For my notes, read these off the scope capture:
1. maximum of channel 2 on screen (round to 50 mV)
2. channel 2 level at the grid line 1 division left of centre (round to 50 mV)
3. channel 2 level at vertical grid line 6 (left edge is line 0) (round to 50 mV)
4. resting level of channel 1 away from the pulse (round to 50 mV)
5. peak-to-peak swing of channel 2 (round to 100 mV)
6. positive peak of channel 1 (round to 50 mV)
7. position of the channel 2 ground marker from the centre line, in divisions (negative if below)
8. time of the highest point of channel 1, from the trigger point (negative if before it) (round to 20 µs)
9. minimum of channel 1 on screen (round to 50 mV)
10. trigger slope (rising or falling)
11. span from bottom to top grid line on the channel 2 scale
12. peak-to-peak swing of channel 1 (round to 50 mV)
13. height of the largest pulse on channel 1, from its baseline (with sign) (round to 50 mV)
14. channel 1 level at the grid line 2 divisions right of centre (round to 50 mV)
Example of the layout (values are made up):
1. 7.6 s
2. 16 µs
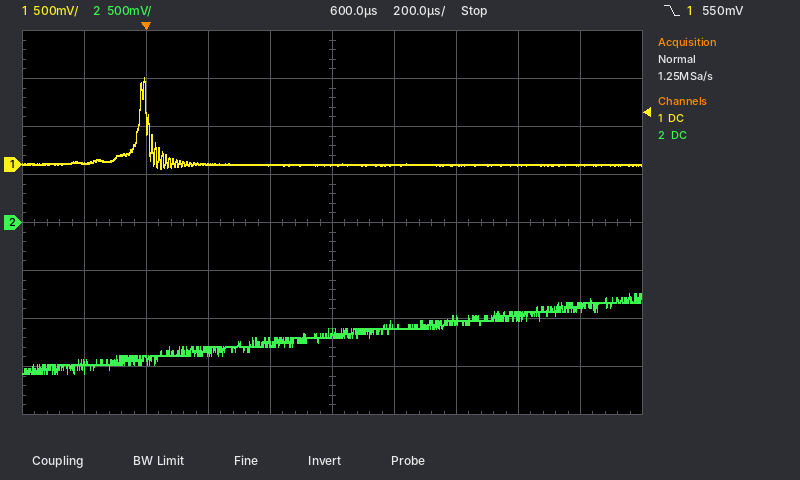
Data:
1. -750 mV
2. -1.25 V
3. -1.10 V
4. 0 mV
5. 800 mV
6. 900 mV
7. 0.0 div
8. 0 µs
9. -50 mV
10. falling
11. 4 V
12. 950 mV
13. +900 mV
14. 0 mV
